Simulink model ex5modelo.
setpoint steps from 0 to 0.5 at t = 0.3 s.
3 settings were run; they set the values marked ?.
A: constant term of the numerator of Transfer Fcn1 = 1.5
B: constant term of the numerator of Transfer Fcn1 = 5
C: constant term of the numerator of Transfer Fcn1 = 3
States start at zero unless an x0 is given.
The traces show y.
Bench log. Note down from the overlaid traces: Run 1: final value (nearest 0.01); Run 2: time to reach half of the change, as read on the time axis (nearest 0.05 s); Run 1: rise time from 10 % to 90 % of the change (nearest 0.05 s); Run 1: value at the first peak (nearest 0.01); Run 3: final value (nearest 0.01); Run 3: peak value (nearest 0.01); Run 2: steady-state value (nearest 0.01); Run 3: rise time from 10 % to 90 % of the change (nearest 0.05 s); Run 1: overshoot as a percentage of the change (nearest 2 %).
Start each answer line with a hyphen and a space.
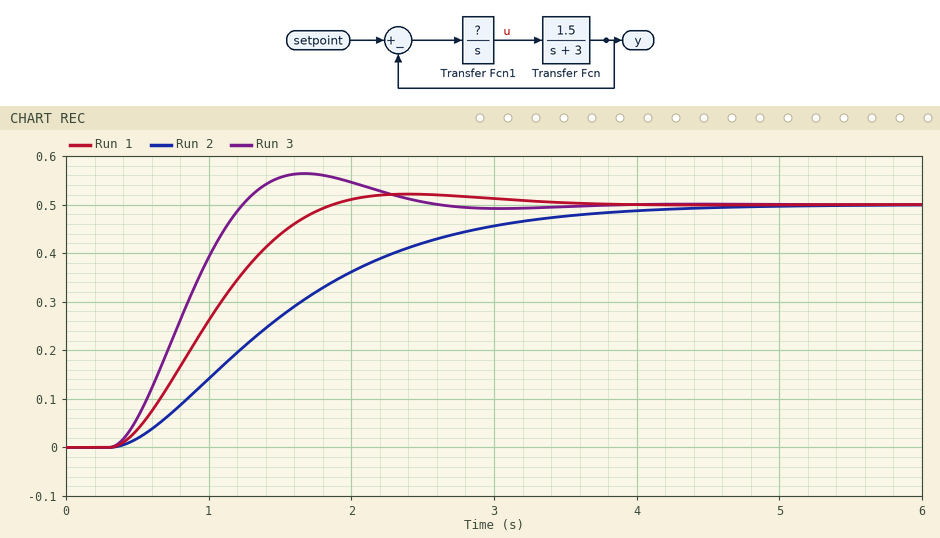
- 0.50
- 1.40 s
- 1.00 s
- 0.52
- 0.50
- 0.56
- 0.50
- 0.65 s
- 4 %
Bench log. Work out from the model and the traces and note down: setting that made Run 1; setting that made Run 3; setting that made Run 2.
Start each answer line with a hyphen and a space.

- C
- B
- A
